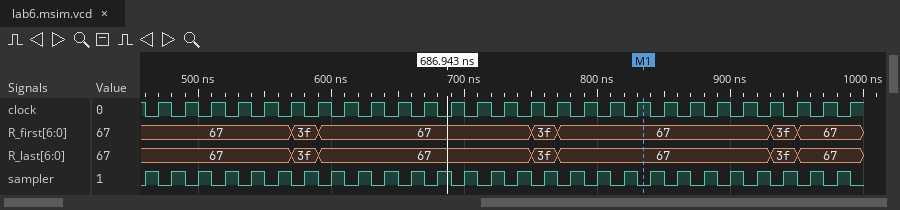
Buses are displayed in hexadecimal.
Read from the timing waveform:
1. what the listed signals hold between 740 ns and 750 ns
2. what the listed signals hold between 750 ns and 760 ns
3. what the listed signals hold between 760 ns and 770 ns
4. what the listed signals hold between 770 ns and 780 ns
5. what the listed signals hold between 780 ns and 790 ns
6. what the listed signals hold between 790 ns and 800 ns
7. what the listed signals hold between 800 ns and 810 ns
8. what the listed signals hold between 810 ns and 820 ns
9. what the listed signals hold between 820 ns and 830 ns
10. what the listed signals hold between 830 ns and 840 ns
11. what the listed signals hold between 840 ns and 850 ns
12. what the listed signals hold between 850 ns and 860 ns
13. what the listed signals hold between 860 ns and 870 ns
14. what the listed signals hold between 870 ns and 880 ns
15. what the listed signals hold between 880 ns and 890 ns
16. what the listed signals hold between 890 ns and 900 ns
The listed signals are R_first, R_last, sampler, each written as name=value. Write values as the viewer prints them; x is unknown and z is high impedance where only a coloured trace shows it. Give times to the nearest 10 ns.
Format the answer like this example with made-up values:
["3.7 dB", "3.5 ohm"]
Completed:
["R_first=67, R_last=67, sampler=1", "R_first=3f, R_last=3f, sampler=0", "R_first=3f, R_last=3f, sampler=1", "R_first=67, R_last=67, sampler=0", "R_first=67, R_last=67, sampler=1", "R_first=67, R_last=67, sampler=0", "R_first=67, R_last=67, sampler=1", "R_first=67, R_last=67, sampler=0", "R_first=67, R_last=67, sampler=1", "R_first=67, R_last=67, sampler=0", "R_first=67, R_last=67, sampler=1", "R_first=67, R_last=67, sampler=0", "R_first=67, R_last=67, sampler=1", "R_first=67, R_last=67, sampler=0", "R_first=67, R_last=67, sampler=1", "R_first=67, R_last=67, sampler=0"]
